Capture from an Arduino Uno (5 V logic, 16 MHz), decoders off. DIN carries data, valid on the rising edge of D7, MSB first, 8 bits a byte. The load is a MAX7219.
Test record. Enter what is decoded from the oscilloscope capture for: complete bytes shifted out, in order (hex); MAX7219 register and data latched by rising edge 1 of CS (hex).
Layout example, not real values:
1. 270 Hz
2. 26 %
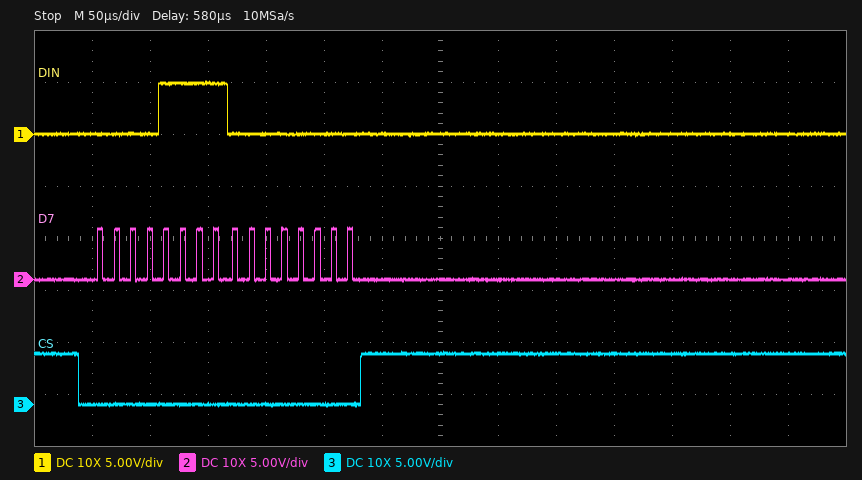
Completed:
1. 0x0F 0x00
2. register 0xF, data 0x00
